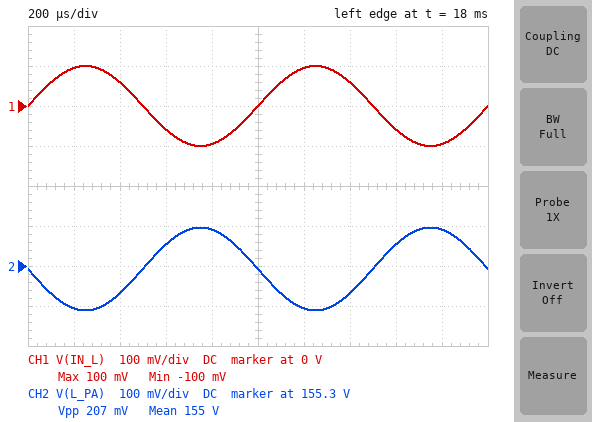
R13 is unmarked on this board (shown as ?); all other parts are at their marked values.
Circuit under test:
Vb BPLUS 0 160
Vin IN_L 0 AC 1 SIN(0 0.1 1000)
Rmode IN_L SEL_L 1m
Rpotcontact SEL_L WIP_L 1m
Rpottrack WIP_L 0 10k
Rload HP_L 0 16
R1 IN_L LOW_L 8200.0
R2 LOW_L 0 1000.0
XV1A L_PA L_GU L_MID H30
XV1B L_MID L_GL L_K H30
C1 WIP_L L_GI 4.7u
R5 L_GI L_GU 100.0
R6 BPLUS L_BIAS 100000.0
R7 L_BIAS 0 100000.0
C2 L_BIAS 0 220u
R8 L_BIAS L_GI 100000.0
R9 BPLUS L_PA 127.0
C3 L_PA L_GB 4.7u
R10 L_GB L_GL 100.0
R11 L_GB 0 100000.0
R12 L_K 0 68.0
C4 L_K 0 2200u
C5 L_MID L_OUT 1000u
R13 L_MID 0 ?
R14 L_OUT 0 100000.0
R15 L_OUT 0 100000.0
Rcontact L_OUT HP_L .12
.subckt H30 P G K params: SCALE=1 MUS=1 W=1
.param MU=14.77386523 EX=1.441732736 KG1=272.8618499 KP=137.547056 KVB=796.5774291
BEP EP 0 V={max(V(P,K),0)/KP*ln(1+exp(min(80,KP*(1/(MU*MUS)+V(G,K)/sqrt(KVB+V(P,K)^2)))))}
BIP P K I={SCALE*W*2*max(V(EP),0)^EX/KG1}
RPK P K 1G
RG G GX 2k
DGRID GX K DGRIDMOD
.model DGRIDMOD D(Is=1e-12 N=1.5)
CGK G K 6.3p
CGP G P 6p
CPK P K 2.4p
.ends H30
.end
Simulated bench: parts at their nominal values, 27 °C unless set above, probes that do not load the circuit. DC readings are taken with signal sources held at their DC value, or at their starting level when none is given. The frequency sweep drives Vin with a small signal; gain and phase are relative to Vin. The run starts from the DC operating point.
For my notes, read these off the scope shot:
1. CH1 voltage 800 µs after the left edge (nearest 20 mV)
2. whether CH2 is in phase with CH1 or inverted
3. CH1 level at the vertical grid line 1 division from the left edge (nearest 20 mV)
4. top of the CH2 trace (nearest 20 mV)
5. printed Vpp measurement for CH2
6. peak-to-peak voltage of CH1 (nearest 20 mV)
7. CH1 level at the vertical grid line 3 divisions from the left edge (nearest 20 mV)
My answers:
-100 mV
inverted
100 mV
155.40 V
207 mV
200 mV
-60 mV
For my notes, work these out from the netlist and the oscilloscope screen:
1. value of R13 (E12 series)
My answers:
150 kΩ
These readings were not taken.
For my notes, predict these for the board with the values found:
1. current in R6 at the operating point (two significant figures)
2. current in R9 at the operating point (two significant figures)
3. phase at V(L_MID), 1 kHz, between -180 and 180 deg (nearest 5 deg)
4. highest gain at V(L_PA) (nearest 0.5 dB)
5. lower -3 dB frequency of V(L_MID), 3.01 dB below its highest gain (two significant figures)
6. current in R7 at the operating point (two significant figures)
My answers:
800 µA
37 mA
0 deg
0.5 dB
280 mHz
800 µA
